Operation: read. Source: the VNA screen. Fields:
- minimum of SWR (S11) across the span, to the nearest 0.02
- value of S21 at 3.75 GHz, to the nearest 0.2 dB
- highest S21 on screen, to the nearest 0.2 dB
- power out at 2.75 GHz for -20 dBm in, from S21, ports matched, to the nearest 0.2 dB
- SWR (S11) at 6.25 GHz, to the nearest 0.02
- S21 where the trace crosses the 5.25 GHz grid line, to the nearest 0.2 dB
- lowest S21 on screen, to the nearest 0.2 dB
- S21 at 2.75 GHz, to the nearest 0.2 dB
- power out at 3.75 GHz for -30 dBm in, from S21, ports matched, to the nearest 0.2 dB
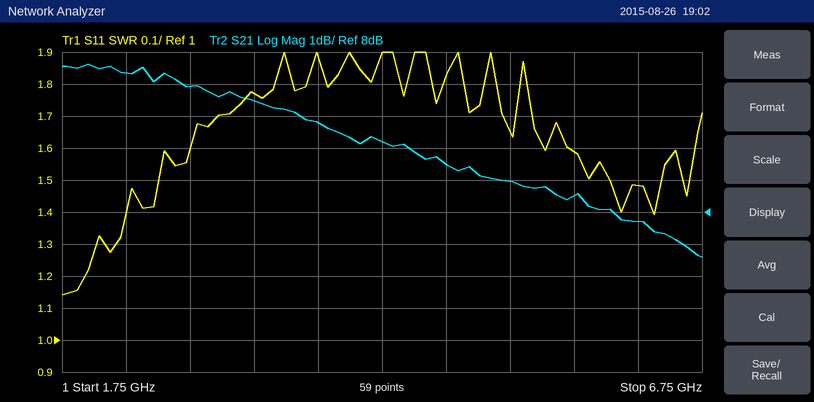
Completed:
1.14
10.8 dB
12.6 dB
-8.0 dBm
1.48
9.0 dB
6.6 dB
12.0 dB
-19.2 dBm
